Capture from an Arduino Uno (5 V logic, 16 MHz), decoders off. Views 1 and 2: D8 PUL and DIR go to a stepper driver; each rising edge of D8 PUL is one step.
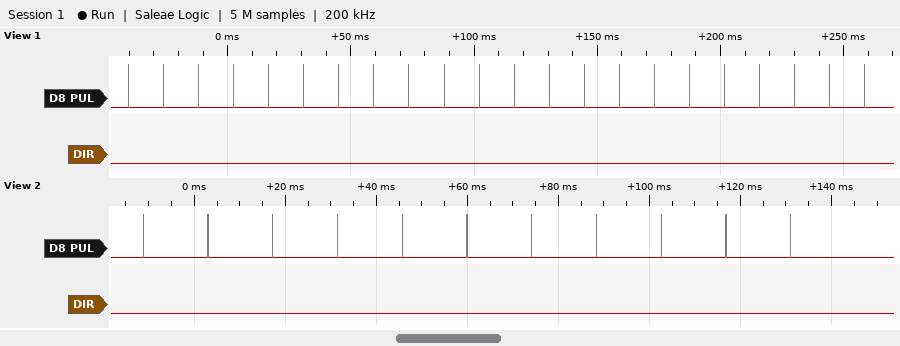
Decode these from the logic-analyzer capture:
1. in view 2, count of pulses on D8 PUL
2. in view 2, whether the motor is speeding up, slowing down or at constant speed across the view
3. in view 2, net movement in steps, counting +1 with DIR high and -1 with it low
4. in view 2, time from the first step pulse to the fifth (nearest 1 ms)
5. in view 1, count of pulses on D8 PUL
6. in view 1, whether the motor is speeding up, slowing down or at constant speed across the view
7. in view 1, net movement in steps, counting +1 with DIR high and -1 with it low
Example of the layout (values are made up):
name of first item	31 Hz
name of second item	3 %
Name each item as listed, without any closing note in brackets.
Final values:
in view 2, count of pulses on D8 PUL	11
in view 2, whether the motor is speeding up, slowing down or at constant speed across the view	constant speed
in view 2, net movement in steps, counting +1 with DIR high and -1 with it low	-11
in view 2, time from the first step pulse to the fifth	57 ms
in view 1, count of pulses on D8 PUL	22
in view 1, whether the motor is speeding up, slowing down or at constant speed across the view	constant speed
in view 1, net movement in steps, counting +1 with DIR high and -1 with it low	-22
